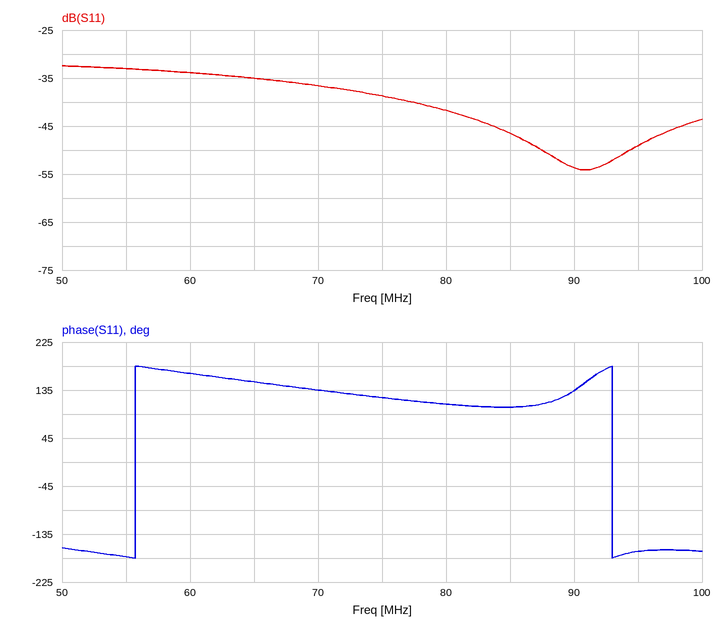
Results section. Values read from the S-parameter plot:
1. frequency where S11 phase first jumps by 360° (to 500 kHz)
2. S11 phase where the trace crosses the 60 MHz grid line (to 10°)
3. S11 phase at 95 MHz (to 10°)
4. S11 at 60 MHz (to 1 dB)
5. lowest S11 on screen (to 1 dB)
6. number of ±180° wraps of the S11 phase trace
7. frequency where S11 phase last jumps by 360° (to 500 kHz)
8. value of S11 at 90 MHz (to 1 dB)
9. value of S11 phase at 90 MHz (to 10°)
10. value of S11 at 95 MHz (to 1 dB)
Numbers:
55.5 MHz
170°
-170°
-34 dB
-54 dB
2
93.0 MHz
-54 dB
130°
-49 dB
